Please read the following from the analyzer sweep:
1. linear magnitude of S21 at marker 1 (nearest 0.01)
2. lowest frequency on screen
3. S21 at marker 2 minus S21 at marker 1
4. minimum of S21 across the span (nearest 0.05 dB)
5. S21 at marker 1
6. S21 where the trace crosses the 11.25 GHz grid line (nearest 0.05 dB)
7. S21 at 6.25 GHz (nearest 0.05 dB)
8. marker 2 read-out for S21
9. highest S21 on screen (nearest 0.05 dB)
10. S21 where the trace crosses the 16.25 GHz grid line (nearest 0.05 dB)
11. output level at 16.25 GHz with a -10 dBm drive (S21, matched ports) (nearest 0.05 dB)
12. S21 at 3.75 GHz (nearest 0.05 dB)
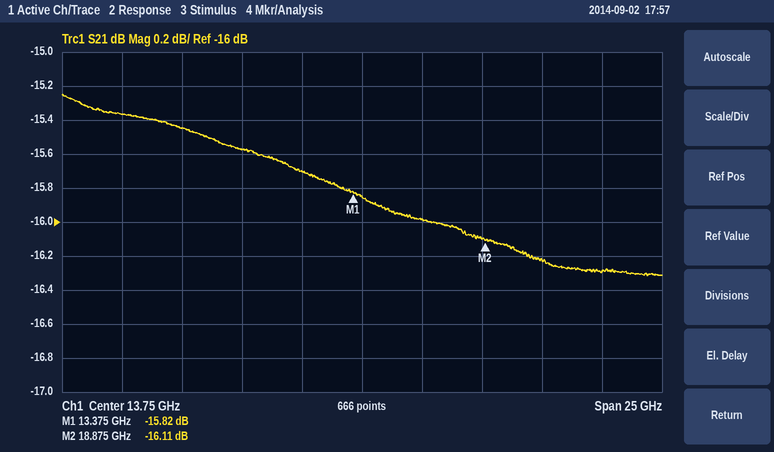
0.16
1.25 GHz
-0.29 dB
-16.30 dB
-15.82 dB
-15.70 dB
-15.45 dB
-16.11 dB
-15.25 dB
-16.00 dB
-26.00 dBm
-15.35 dB
